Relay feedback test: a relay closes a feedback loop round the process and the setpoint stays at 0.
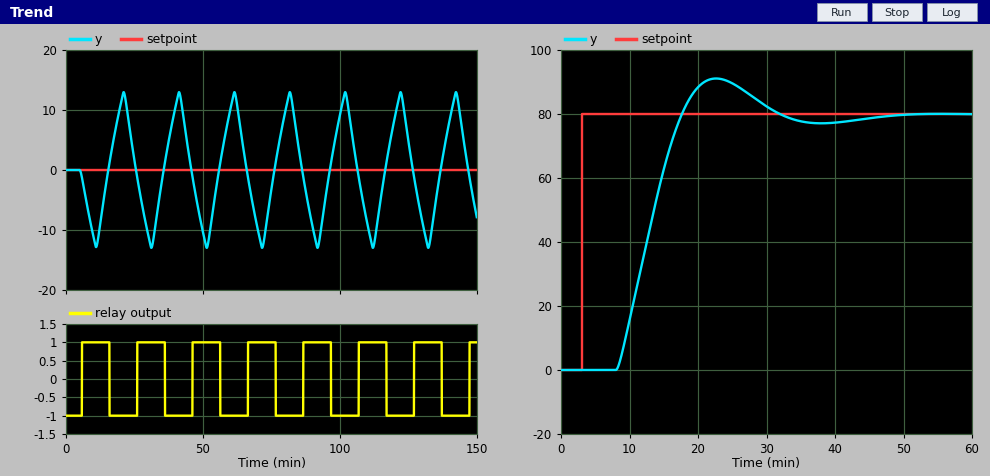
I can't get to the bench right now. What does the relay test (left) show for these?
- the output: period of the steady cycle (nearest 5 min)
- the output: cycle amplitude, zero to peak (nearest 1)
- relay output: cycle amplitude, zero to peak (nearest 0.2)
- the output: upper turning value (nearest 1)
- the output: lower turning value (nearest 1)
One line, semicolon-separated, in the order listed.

20 min; 13; 1.0; 13; -13
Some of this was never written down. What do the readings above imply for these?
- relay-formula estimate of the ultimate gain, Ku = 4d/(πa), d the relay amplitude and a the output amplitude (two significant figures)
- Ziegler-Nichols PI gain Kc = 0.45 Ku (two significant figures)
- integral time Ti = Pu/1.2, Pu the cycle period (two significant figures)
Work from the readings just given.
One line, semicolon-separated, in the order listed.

0.098; 0.044; 17 min
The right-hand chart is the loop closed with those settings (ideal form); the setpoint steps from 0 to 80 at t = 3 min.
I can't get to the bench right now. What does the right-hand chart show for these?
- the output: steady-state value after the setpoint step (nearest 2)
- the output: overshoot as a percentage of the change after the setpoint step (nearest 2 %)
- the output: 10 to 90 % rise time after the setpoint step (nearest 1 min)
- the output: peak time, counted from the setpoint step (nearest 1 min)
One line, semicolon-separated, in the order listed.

80; 14 %; 7 min; 20 min
